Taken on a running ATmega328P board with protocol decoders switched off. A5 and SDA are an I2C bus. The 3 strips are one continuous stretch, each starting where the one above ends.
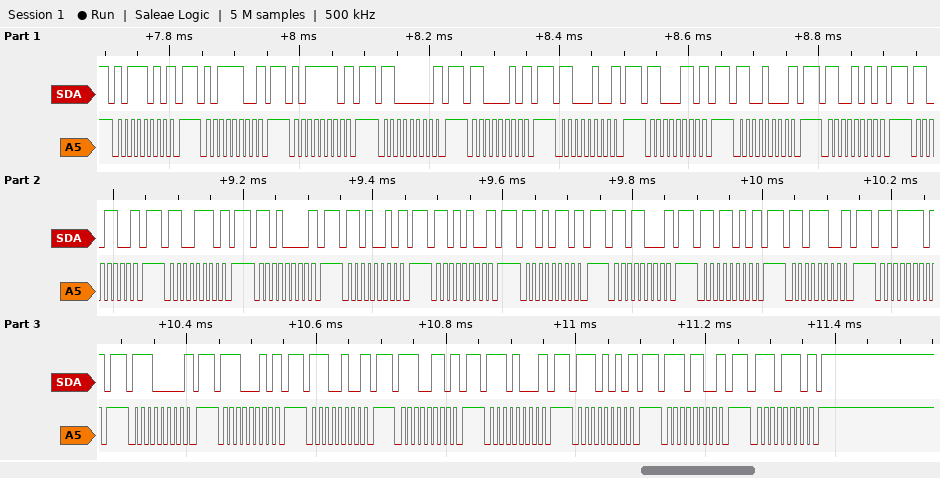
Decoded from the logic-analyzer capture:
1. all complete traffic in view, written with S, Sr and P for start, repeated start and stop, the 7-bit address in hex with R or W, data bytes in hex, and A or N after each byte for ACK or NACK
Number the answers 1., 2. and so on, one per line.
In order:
1. S 5DW N P S 5EW N P S 5FW N P S 60W N P S 61W N P S 62W N P S 63W N P S 64W N P S 65W N P S 66W N P S 67W N P S 68W N P S 69W N P S 6AW N P S 6BW N P S 6CW N P S 6DW N P S 6EW N P S 6FW N P S 70W N P S 71W N P S 72W N P S 73W N P S 74W N P S 75W N P S 76W N P S 77W N P
